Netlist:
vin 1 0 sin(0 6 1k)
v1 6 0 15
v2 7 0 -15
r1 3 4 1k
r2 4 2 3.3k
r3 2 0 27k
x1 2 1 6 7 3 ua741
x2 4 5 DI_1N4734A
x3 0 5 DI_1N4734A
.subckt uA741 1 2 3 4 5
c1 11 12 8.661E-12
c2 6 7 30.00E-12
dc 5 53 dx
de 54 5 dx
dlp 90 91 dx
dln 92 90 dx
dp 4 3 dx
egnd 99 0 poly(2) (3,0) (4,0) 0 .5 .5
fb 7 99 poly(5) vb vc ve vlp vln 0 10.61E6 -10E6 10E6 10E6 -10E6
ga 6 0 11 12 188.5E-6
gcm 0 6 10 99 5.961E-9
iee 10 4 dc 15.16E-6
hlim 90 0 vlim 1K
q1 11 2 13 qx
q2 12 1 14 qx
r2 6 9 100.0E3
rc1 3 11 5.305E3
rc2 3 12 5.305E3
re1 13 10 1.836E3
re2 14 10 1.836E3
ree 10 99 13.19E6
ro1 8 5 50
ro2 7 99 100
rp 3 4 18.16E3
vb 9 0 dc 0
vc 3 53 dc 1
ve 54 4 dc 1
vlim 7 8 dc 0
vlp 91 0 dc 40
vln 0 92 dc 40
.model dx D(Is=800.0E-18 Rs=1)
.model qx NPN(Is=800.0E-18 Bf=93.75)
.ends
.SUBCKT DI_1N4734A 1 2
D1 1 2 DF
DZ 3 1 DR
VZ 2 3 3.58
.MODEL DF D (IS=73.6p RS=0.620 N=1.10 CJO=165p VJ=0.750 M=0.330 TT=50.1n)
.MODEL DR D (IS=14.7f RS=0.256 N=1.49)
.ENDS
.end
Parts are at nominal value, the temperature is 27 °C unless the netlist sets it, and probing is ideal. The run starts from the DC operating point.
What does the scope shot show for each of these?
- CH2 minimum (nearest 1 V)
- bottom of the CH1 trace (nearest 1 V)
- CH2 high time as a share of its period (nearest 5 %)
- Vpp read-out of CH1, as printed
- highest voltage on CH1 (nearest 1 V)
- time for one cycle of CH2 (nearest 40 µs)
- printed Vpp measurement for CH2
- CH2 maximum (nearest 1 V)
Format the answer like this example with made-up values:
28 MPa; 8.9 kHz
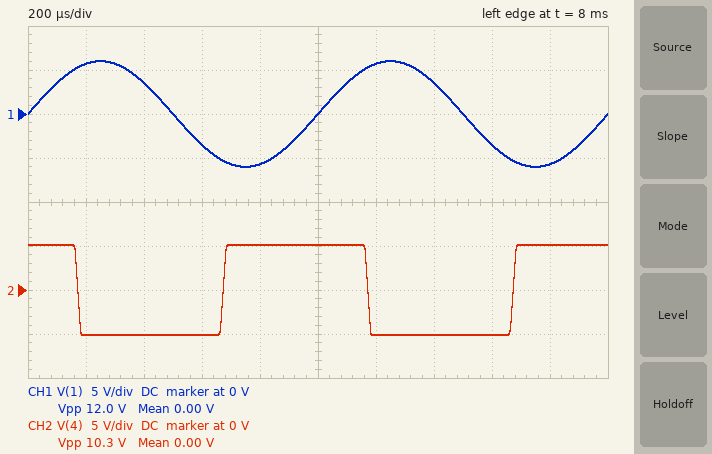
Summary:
-5 V; -6 V; 50 %; 12.0 V; 6 V; 1.00 ms; 10.3 V; 5 V
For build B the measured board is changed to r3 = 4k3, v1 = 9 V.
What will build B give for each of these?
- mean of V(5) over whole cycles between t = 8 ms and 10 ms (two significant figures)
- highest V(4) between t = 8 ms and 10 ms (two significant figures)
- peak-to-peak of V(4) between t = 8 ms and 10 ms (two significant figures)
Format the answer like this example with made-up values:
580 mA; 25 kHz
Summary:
1.9 V; 5.1 V; 10 V
